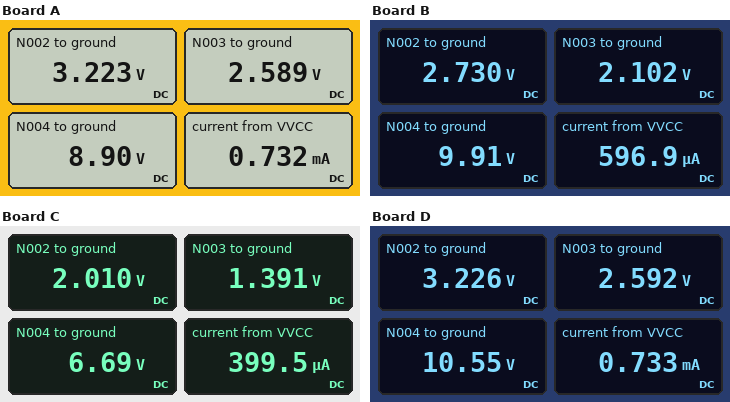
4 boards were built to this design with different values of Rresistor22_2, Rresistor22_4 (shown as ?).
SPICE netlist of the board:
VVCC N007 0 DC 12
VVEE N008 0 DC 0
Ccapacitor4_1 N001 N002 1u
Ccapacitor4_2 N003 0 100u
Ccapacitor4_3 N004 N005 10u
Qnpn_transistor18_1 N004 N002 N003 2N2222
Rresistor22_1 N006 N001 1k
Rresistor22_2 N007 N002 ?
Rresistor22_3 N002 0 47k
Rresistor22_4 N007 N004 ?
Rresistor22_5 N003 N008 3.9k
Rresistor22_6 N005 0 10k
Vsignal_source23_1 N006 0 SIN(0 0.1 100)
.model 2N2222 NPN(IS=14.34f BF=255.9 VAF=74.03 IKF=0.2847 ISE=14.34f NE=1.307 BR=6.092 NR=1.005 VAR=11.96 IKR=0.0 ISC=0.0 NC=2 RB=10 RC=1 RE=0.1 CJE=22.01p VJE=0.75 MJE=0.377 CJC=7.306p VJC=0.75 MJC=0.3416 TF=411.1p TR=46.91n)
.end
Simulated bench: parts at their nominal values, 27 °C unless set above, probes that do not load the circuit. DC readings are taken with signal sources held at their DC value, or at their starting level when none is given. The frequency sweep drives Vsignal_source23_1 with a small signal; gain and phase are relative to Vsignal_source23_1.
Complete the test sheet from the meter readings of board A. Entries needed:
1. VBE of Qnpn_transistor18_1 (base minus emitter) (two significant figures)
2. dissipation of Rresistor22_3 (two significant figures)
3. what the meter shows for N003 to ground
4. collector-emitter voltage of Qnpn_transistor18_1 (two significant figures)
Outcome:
630 mV
220 µW
2.589 V
6.3 V
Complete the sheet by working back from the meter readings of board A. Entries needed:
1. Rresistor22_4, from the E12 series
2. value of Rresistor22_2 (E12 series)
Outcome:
4.7 kΩ
120 kΩ
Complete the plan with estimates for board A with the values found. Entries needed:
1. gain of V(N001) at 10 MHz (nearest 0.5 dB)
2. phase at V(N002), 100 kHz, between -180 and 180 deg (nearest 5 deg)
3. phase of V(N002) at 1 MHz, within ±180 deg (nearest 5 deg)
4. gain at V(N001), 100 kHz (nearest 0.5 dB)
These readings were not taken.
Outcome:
-24.0 dB
-10 deg
-55 deg
-1.5 dB
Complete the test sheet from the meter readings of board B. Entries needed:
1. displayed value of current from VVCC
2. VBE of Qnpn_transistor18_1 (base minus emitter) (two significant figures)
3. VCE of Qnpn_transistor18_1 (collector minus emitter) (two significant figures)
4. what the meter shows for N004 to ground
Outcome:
596.9 µA
630 mV
7.8 V
9.91 V
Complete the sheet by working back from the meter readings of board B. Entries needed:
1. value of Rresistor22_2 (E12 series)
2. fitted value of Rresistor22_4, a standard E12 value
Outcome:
150 kΩ
3.9 kΩ
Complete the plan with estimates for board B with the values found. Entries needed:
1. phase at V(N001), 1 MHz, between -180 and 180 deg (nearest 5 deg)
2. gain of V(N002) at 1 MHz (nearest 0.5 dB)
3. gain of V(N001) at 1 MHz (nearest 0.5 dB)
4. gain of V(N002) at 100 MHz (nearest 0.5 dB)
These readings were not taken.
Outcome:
-50 deg
-5.5 dB
-5.5 dB
-30.0 dB
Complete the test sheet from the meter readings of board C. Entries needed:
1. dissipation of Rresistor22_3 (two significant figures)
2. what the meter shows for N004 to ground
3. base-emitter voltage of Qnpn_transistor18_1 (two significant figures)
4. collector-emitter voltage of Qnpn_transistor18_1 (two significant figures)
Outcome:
86 µW
6.69 V
620 mV
5.3 V
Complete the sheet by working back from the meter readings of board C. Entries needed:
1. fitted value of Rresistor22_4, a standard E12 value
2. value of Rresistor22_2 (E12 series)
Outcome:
15 kΩ
220 kΩ
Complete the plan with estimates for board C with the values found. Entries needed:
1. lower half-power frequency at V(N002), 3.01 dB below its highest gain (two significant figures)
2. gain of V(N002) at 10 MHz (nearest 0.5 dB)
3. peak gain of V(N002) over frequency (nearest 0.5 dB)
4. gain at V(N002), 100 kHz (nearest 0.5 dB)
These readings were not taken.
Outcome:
16 Hz
-22.0 dB
-1.0 dB
-1.0 dB
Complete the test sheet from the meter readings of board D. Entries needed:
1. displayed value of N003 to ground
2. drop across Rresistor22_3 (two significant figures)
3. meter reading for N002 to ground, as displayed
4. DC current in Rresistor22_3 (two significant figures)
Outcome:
2.592 V
3.2 V
3.226 V
69 µA
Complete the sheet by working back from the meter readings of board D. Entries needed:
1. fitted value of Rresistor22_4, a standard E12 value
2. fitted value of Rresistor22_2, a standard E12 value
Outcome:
2.2 kΩ
120 kΩ
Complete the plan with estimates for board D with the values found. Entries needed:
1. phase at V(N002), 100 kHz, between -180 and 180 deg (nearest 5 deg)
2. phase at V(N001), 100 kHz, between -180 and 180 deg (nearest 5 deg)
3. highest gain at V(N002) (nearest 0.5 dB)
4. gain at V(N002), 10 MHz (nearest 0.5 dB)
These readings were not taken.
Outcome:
-5 deg
-5 deg
-1.5 dB
-21.5 dB
